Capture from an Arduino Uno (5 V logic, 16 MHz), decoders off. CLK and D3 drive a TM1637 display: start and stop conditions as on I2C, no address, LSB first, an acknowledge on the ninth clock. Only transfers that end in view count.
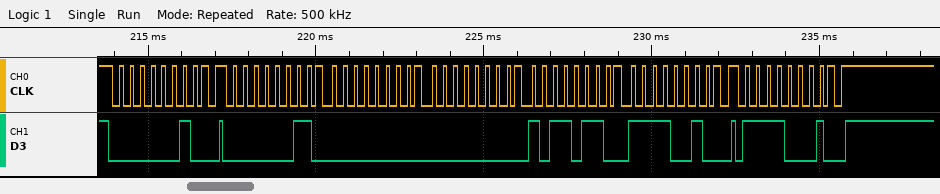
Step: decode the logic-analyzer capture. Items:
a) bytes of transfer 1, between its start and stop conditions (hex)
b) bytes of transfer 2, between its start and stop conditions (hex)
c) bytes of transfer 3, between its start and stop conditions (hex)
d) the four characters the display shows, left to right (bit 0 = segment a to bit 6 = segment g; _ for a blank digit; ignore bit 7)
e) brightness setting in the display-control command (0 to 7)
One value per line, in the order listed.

40
C0 00 00 6D 4F
8F
__53
7
